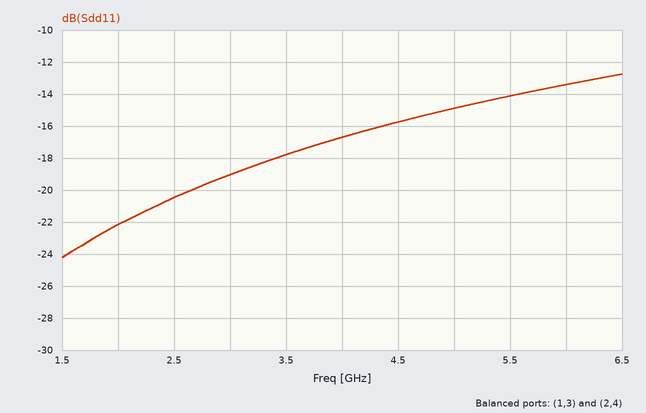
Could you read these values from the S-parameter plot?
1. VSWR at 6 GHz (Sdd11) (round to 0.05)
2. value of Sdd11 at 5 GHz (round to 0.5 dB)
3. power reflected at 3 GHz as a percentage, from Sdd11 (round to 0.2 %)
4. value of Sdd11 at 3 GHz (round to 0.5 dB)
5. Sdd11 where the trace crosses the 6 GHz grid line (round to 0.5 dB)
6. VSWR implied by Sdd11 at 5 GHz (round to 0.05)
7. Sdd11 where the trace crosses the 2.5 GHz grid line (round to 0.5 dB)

1.55
-15.0 dB
1.2 %
-19.0 dB
-13.5 dB
1.45
-20.5 dB
